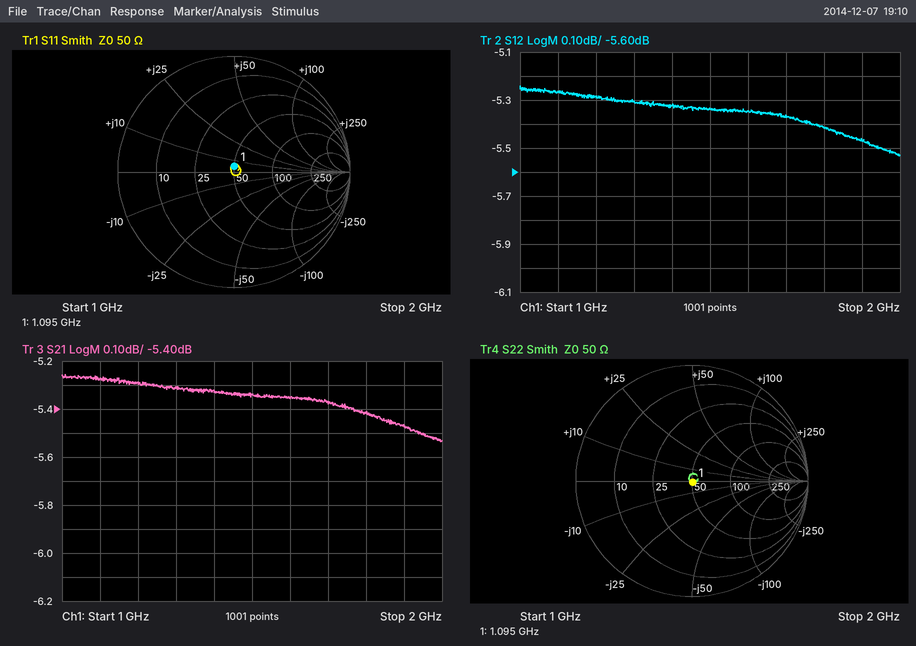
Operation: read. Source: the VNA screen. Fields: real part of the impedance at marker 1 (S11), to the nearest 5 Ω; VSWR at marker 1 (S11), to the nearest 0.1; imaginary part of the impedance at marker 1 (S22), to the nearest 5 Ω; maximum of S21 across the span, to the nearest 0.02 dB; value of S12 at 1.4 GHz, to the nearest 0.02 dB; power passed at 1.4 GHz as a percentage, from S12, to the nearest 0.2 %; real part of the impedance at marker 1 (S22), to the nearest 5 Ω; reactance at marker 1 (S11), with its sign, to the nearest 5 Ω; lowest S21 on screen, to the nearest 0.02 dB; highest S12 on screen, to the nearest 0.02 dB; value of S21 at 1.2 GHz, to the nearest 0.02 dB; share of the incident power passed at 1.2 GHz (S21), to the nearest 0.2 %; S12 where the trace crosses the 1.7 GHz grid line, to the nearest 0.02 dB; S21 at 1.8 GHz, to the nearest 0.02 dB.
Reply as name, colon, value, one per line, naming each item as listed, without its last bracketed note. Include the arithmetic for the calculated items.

real part of the impedance at marker 1 (S11), to the nearest 5 Ω: 50 Ω
VSWR at marker 1 (S11), to the nearest 0.1: 1.1
imaginary part of the impedance at marker 1 (S22), to the nearest 5 Ω: 0 Ω
maximum of S21 across the span, to the nearest 0.02 dB: -5.26 dB
value of S12 at 1.4 GHz, to the nearest 0.02 dB: -5.32 dB
power passed at 1.4 GHz as a percentage, from S12, to the nearest 0.2 %: 10^(-5.32/10) ≈ 29.4 %
real part of the impedance at marker 1 (S22), to the nearest 5 Ω: 50 Ω
reactance at marker 1 (S11), with its sign, to the nearest 5 Ω: +5 Ω
lowest S21 on screen, to the nearest 0.02 dB: -5.54 dB
highest S12 on screen, to the nearest 0.02 dB: -5.24 dB
value of S21 at 1.2 GHz, to the nearest 0.02 dB: -5.30 dB
share of the incident power passed at 1.2 GHz (S21), to the nearest 0.2 %: 10^(-5.3/10) ≈ 29.5 %, so 29.6 % to the nearest 0.2 %
S12 where the trace crosses the 1.7 GHz grid line, to the nearest 0.02 dB: -5.36 dB
S21 at 1.8 GHz, to the nearest 0.02 dB: -5.42 dB
